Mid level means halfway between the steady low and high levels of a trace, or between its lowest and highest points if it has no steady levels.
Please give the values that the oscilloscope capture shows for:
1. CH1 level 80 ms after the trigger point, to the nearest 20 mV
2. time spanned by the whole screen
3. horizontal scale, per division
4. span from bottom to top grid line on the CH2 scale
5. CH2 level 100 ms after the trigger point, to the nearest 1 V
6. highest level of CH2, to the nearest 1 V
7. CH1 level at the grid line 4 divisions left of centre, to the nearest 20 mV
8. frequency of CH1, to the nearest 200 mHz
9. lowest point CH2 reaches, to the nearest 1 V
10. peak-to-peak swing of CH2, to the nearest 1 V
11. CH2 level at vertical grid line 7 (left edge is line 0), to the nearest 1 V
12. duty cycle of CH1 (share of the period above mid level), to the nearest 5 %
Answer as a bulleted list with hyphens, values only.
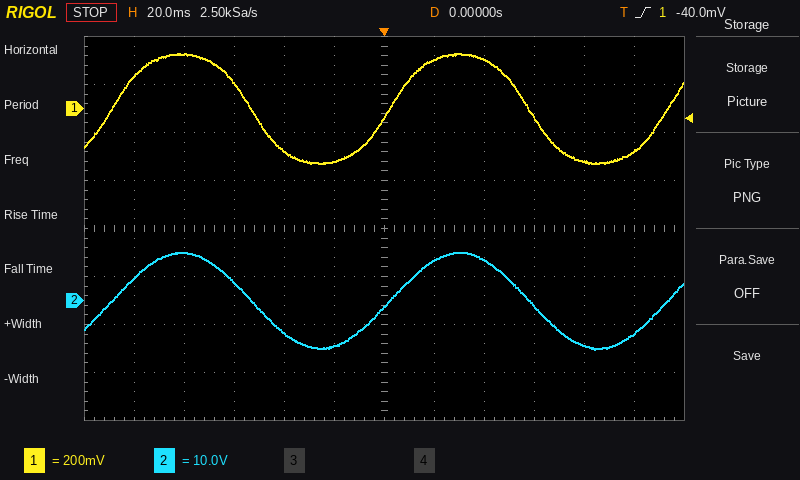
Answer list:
- -220 mV
- 240 ms
- 20 ms
- 80 V
- -7 V
- 10 V
- 220 mV
- 9.0 Hz
- -10 V
- 20 V
- 8 V
- 50 %
